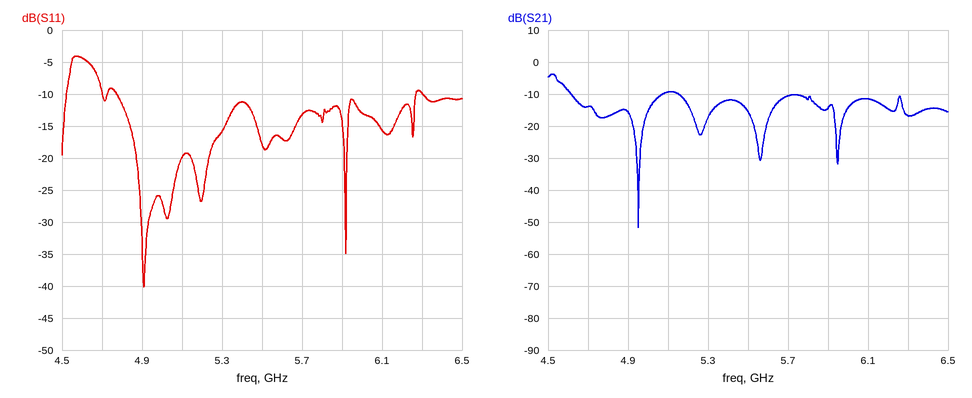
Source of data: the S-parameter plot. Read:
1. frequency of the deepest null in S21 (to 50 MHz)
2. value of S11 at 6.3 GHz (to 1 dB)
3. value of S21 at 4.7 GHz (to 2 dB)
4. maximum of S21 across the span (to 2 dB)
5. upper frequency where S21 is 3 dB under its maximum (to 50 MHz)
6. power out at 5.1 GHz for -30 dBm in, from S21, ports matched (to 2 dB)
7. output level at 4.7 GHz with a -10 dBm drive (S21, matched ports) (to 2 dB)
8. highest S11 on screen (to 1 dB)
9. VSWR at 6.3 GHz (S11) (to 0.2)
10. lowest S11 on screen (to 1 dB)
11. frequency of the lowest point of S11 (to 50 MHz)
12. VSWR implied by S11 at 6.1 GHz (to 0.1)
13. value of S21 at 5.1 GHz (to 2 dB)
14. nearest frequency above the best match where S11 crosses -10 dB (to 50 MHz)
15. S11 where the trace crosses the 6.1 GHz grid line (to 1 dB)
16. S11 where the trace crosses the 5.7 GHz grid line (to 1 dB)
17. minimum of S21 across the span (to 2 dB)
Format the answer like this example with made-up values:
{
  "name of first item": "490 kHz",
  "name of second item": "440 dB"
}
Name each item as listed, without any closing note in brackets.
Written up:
{
  "frequency of the deepest null in S21": "4.95 GHz",
  "value of S11 at 6.3 GHz": "-10 dB",
  "value of S21 at 4.7 GHz": "-14 dB",
  "maximum of S21 across the span": "-4 dB",
  "upper frequency where S21 is 3 dB under its maximum": "4.55 GHz",
  "power out at 5.1 GHz for -30 dBm in, from S21, ports matched": "-40 dBm",
  "output level at 4.7 GHz with a -10 dBm drive (S21, matched ports)": "-24 dBm",
  "highest S11 on screen": "-4 dB",
  "VSWR at 6.3 GHz (S11)": "2.0",
  "lowest S11 on screen": "-40 dB",
  "frequency of the lowest point of S11": "4.90 GHz",
  "VSWR implied by S11 at 6.1 GHz": "1.4",
  "value of S21 at 5.1 GHz": "-10 dB",
  "nearest frequency above the best match where S11 crosses -10 dB": "6.25 GHz",
  "S11 where the trace crosses the 6.1 GHz grid line": "-16 dB",
  "S11 where the trace crosses the 5.7 GHz grid line": "-13 dB",
  "minimum of S21 across the span": "-52 dB"
}
